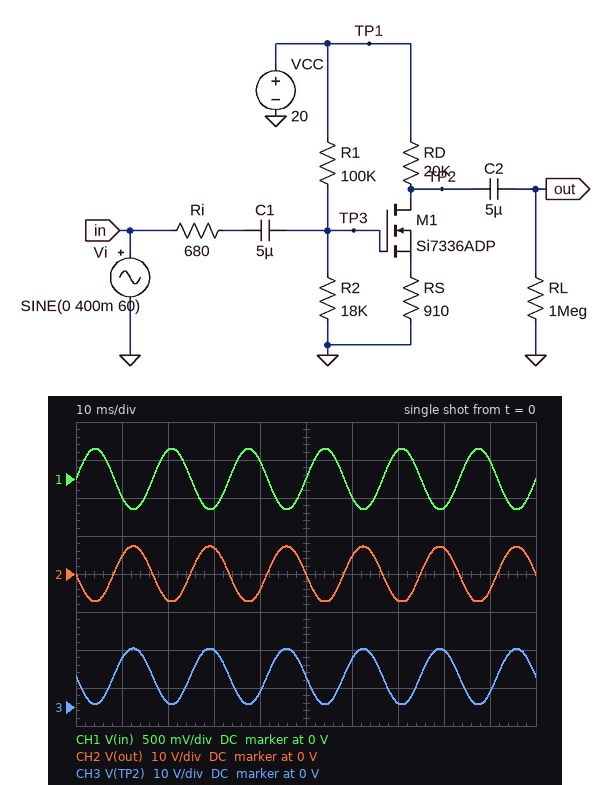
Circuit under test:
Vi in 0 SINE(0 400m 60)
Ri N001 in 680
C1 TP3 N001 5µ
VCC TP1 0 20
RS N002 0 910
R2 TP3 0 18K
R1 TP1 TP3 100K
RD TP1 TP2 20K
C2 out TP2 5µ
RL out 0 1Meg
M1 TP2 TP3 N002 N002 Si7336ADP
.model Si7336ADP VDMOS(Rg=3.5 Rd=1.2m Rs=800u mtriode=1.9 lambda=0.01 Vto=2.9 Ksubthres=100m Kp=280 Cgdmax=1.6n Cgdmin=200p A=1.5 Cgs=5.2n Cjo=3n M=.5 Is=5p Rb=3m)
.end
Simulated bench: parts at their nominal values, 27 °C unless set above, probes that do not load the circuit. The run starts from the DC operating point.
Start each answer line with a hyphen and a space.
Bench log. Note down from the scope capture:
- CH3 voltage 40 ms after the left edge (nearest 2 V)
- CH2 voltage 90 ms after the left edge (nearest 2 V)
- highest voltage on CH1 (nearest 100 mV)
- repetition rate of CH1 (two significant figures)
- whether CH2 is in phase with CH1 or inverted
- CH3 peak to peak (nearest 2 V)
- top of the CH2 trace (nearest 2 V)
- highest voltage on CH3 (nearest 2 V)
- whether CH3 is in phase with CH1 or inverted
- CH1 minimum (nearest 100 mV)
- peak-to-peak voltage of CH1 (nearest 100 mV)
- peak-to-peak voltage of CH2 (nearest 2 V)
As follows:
- 4 V
- -4 V
- 400 mV
- 60 Hz
- inverted
- 14 V
- 8 V
- 16 V
- inverted
- -400 mV
- 800 mV
- 14 V
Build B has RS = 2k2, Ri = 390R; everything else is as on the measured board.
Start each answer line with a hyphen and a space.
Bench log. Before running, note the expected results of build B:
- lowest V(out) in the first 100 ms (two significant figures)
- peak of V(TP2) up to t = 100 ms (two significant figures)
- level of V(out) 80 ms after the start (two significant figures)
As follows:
- -3.2 V
- 18 V
- 2.9 V
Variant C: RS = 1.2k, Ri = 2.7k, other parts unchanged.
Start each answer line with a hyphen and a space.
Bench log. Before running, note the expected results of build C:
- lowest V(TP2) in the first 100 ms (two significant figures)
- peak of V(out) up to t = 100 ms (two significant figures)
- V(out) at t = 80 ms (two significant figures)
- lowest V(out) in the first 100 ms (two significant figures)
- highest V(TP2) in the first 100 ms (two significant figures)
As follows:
- 5.7 V
- 5.0 V
- 4.7 V
- -5.1 V
- 16 V
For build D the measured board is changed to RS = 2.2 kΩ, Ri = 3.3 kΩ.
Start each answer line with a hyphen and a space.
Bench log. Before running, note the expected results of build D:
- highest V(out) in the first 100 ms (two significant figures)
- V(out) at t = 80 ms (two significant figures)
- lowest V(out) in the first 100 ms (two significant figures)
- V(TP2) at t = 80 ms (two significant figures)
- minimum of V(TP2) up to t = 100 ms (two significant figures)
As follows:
- 2.7 V
- 2.5 V
- -2.7 V
- 17 V
- 12 V
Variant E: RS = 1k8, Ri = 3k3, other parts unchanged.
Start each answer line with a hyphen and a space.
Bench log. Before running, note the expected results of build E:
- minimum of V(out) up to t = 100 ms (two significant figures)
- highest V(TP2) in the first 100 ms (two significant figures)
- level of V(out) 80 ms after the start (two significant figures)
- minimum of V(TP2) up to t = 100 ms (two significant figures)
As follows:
- -3.3 V
- 17 V
- 3.0 V
- 10 V
